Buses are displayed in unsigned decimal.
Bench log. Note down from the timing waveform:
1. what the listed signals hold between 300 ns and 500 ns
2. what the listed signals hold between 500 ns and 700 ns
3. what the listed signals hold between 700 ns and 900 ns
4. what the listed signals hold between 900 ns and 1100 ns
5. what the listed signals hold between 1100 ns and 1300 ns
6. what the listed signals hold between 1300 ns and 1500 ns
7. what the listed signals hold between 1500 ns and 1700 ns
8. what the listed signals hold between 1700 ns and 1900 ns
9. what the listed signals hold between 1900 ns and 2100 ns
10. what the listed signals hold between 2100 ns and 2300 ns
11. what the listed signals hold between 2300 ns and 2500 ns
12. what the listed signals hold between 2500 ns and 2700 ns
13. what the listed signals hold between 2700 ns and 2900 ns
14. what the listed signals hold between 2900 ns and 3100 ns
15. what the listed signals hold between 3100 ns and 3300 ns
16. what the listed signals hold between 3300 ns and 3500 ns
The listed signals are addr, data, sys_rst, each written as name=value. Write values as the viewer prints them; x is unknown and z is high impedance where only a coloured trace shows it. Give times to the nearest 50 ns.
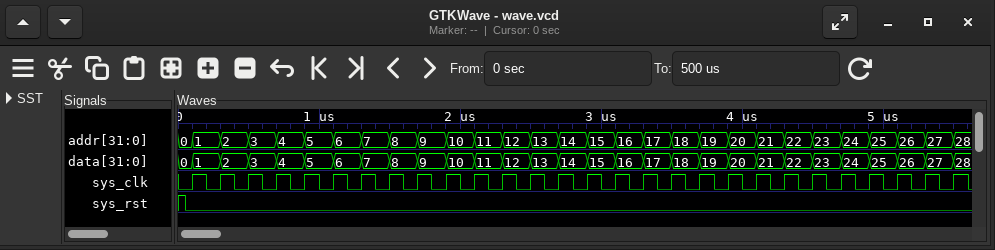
addr=2, data=2, sys_rst=0
addr=3, data=3, sys_rst=0
addr=4, data=4, sys_rst=0
addr=5, data=5, sys_rst=0
addr=6, data=6, sys_rst=0
addr=7, data=7, sys_rst=0
addr=8, data=8, sys_rst=0
addr=9, data=9, sys_rst=0
addr=10, data=10, sys_rst=0
addr=11, data=11, sys_rst=0
addr=12, data=12, sys_rst=0
addr=13, data=13, sys_rst=0
addr=14, data=14, sys_rst=0
addr=15, data=15, sys_rst=0
addr=16, data=16, sys_rst=0
addr=17, data=17, sys_rst=0
